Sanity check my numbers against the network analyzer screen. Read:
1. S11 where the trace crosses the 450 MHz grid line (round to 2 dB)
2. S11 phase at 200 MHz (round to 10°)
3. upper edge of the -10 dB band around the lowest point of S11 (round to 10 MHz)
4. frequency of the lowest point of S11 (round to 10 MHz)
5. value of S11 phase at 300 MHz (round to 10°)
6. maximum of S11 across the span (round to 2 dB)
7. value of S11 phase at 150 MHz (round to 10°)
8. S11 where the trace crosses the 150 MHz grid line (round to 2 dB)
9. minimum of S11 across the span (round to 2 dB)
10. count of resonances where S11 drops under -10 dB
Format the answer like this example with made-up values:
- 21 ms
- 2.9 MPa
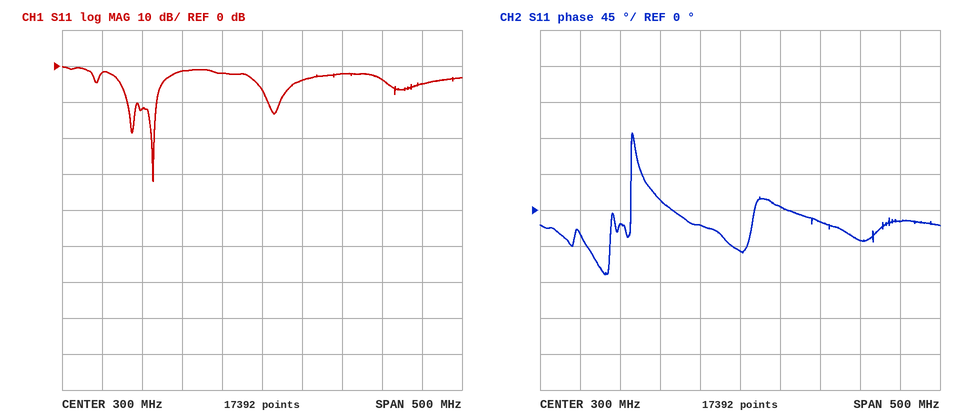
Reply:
- -4 dB
- 10°
- 170 MHz
- 160 MHz
- -50°
- 0 dB
- -20°
- -12 dB
- -32 dB
- 3
